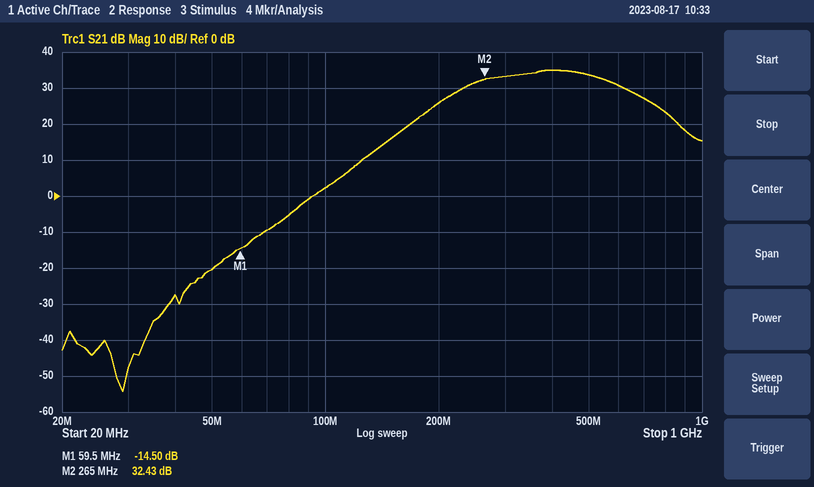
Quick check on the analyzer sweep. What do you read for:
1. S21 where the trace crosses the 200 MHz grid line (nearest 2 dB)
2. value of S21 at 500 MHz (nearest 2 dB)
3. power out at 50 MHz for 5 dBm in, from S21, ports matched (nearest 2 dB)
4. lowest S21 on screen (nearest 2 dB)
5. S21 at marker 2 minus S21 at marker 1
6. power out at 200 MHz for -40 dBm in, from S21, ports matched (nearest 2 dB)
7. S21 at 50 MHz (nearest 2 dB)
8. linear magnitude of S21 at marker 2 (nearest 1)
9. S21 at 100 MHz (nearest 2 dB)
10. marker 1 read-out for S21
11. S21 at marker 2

26 dB
34 dB
-16 dBm
-54 dB
46.93 dB
-14 dBm
-20 dB
42
2 dB
-14.50 dB
32.43 dB
